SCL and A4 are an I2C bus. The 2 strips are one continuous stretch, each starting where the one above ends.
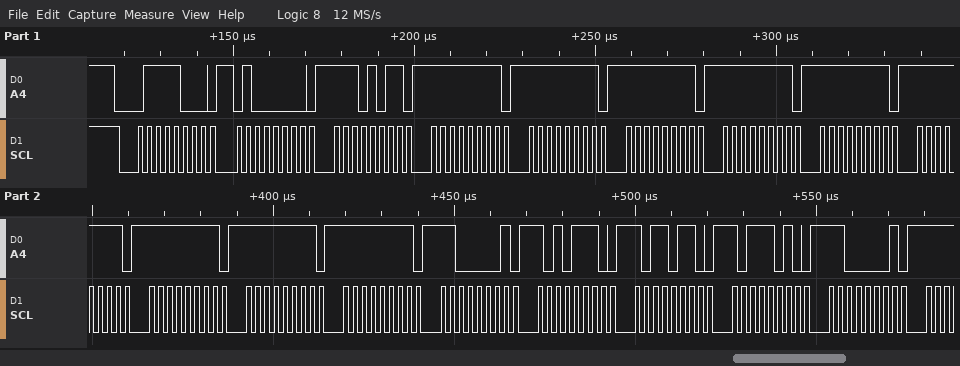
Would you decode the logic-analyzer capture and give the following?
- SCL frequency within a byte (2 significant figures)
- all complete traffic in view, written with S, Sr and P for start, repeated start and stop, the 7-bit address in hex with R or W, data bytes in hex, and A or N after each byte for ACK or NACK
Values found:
400 kHz
S 3CW A 40 A EB A FF A FF A FF A FF A FF A FF A FF A FF A FF A C1 A AE A B6 A BA A C1 A
